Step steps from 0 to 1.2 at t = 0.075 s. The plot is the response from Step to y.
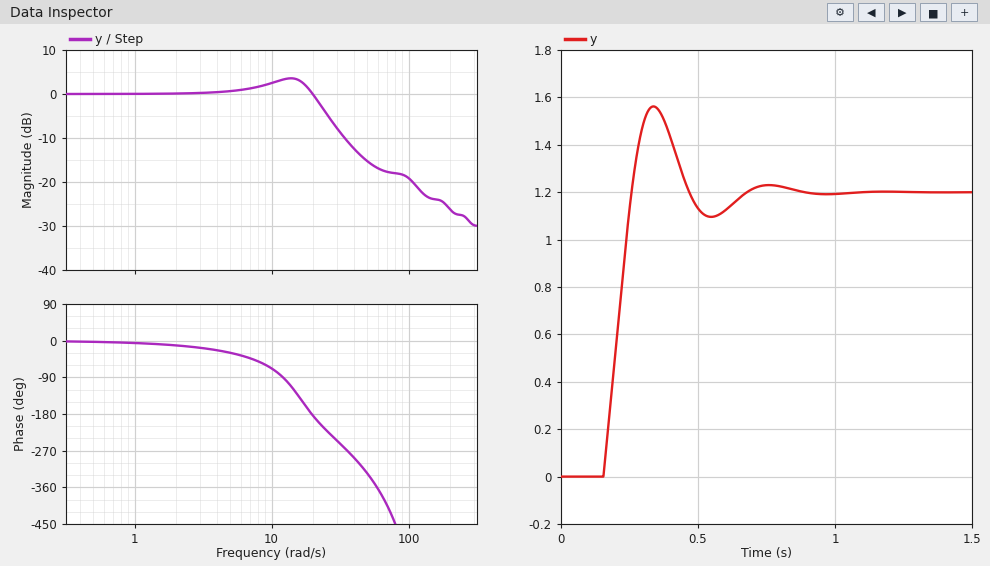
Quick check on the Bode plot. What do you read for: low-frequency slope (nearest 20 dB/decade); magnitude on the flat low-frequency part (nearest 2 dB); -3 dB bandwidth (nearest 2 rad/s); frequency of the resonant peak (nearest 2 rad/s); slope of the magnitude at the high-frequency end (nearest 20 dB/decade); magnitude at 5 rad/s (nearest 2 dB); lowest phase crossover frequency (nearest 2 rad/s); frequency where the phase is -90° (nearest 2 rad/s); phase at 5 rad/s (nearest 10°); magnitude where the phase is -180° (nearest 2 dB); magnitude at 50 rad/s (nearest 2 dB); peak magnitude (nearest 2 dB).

0 dB/decade
0 dB
24 rad/s
14 rad/s
-20 dB/decade
0 dB
20 rad/s
12 rad/s
-30°
0 dB
-16 dB
4 dB
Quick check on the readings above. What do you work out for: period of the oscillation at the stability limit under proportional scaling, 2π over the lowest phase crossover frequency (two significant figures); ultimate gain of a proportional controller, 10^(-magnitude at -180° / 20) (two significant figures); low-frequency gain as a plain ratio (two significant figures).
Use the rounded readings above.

0.31 s
1.0
1.0
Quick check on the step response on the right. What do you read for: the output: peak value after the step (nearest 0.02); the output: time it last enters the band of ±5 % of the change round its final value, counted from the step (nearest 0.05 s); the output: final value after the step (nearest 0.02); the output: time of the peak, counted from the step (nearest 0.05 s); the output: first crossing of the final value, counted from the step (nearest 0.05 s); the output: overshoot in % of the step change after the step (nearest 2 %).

1.56
0.55 s
1.20
0.25 s
0.20 s
30 %
